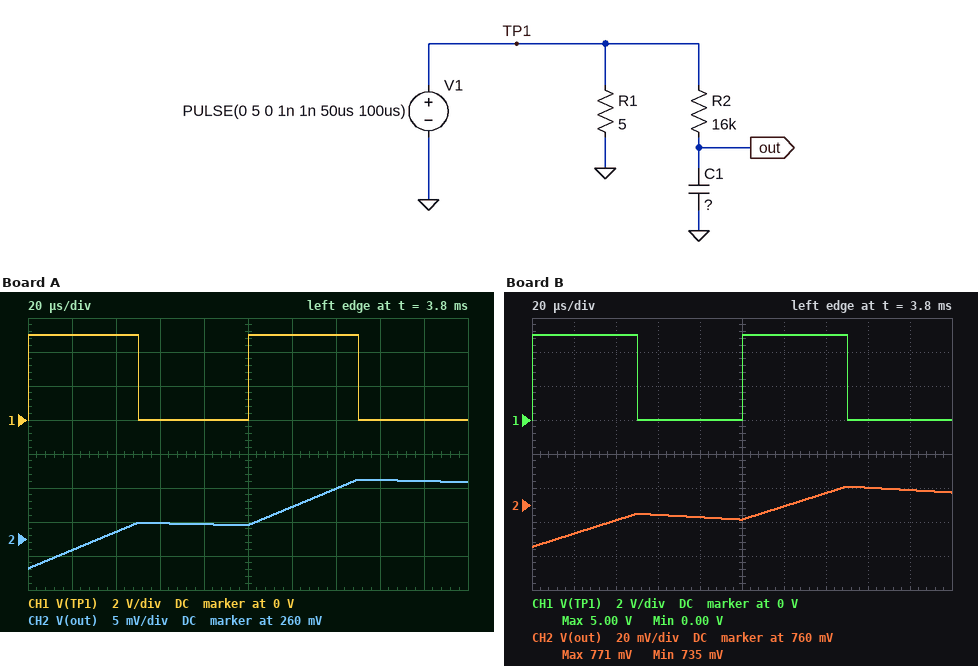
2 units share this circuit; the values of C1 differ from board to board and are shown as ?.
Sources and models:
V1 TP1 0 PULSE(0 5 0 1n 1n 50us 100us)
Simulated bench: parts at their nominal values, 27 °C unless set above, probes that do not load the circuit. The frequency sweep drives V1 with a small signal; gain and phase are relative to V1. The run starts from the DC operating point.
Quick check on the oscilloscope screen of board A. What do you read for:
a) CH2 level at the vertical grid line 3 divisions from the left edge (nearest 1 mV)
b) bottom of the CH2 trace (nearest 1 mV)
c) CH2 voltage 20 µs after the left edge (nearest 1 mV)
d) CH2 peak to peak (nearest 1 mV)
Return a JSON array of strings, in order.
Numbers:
["262 mV", "256 mV", "258 mV", "13 mV"]
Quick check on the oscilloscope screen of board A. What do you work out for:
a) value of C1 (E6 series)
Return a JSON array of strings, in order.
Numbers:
["2.2 µF"]
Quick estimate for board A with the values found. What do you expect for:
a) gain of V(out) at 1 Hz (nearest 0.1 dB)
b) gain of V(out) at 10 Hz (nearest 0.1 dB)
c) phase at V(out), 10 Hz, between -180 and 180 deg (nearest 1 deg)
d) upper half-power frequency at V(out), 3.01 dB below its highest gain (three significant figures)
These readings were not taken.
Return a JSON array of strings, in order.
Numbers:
["-0.2 dB", "-7.7 dB", "-66 deg", "4.52 Hz"]
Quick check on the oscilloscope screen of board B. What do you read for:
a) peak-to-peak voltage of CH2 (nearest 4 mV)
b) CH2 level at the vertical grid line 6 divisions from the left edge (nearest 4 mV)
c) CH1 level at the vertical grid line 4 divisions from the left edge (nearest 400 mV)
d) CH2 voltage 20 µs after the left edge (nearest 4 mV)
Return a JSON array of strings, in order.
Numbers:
["36 mV", "760 mV", "0 V", "744 mV"]
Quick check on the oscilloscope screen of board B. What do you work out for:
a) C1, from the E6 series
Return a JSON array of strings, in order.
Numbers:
["680 nF"]
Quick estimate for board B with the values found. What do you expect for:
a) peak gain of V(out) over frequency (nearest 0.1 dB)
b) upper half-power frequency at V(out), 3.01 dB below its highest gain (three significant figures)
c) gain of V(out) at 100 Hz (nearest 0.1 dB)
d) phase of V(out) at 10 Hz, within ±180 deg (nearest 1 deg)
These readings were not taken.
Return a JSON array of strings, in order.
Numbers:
["0 dB", "14.6 Hz", "-16.8 dB", "-34 deg"]
